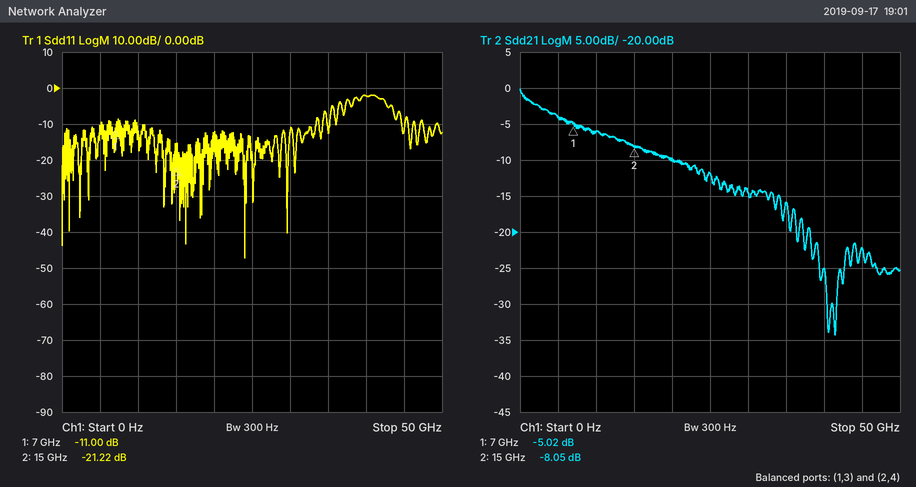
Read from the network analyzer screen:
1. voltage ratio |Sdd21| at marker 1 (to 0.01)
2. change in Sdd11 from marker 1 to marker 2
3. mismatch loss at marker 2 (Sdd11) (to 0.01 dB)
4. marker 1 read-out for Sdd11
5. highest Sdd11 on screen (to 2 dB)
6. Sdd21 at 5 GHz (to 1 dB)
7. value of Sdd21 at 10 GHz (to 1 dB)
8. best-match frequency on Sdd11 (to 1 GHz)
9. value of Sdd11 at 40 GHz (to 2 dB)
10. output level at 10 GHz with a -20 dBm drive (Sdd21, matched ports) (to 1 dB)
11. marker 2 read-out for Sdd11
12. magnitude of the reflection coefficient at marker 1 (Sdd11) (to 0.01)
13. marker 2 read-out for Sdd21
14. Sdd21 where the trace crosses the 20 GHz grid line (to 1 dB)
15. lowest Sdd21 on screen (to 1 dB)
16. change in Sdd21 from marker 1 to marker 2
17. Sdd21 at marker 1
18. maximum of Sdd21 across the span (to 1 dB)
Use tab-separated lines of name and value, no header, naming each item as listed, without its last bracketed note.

voltage ratio |Sdd21| at marker 1	0.56
change in Sdd11 from marker 1 to marker 2	-10.22 dB
mismatch loss at marker 2 (Sdd11)	0.03 dB
marker 1 read-out for Sdd11	-11.00 dB
highest Sdd11 on screen	-2 dB
Sdd21 at 5 GHz	-4 dB
value of Sdd21 at 10 GHz	-6 dB
best-match frequency on Sdd11	24 GHz
value of Sdd11 at 40 GHz	-2 dB
output level at 10 GHz with a -20 dBm drive (Sdd21, matched ports)	-26 dBm
marker 2 read-out for Sdd11	-21.22 dB
magnitude of the reflection coefficient at marker 1 (Sdd11)	0.28
marker 2 read-out for Sdd21	-8.05 dB
Sdd21 where the trace crosses the 20 GHz grid line	-10 dB
lowest Sdd21 on screen	-34 dB
change in Sdd21 from marker 1 to marker 2	-3.03 dB
Sdd21 at marker 1	-5.02 dB
maximum of Sdd21 across the span	0 dB
